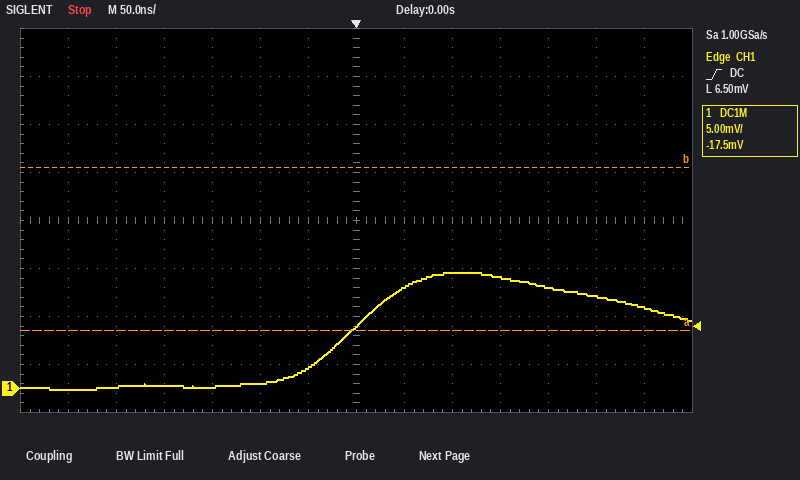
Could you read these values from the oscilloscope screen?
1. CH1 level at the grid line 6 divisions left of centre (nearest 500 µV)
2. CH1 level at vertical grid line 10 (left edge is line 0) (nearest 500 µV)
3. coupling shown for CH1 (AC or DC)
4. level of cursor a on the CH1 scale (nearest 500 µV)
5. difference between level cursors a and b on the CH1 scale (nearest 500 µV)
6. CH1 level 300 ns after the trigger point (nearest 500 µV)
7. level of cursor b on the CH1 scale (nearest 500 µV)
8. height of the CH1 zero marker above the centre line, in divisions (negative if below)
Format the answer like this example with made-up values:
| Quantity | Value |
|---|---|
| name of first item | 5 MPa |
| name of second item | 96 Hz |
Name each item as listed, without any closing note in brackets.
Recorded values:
| Quantity | Value |
|---|---|
| CH1 level at the grid line 6 divisions left of centre | 0.0 mV |
| CH1 level at vertical grid line 10 (left edge is line 0) | 11.5 mV |
| coupling shown for CH1 | DC |
| level of cursor a on the CH1 scale | 6.0 mV |
| difference between level cursors a and b on the CH1 scale | 17.0 mV |
| CH1 level 300 ns after the trigger point | 8.5 mV |
| level of cursor b on the CH1 scale | 23.0 mV |
| height of the CH1 zero marker above the centre line, in divisions | -3.5 div |
